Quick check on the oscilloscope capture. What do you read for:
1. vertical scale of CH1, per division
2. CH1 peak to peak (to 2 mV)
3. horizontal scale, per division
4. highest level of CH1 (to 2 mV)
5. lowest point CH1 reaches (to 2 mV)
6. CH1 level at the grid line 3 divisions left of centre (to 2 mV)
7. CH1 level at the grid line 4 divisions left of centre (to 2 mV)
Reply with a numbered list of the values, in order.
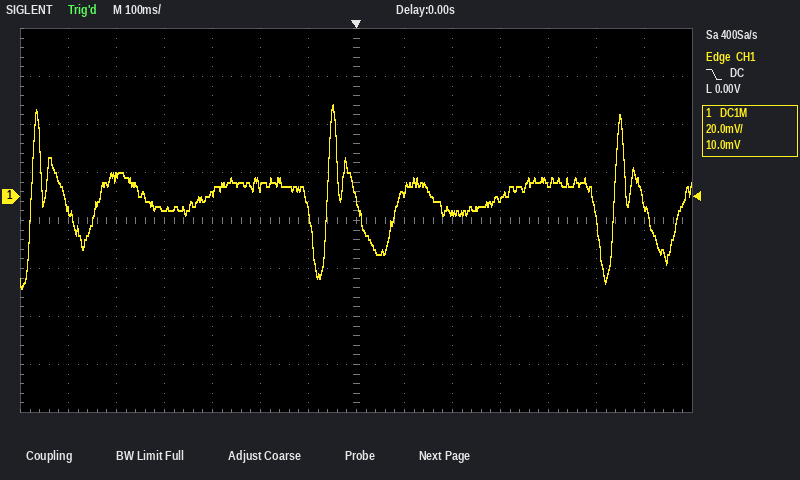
1. 20 mV
2. 76 mV
3. 100 ms
4. 38 mV
5. -38 mV
6. 2 mV
7. -6 mV
